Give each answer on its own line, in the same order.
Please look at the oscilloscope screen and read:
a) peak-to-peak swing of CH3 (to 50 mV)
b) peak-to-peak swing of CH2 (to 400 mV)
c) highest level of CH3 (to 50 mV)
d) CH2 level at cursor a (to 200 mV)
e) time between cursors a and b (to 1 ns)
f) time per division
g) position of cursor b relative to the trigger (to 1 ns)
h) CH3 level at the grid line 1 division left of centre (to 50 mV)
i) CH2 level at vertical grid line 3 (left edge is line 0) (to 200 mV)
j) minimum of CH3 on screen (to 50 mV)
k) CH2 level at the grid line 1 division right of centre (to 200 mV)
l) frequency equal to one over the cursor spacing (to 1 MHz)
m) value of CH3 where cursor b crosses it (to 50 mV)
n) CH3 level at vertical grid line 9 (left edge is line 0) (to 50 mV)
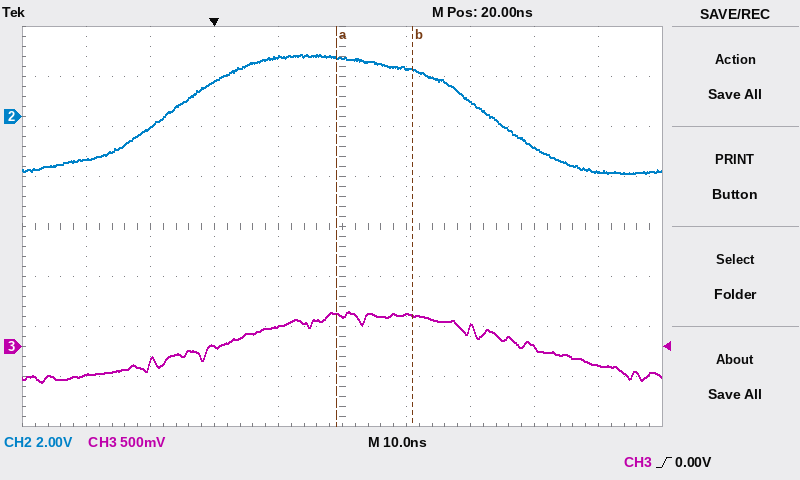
700 mV
4.8 V
350 mV
2.4 V
12 ns
10 ns
+31 ns
200 mV
1.4 V
-350 mV
2.0 V
83 MHz
300 mV
-200 mV
